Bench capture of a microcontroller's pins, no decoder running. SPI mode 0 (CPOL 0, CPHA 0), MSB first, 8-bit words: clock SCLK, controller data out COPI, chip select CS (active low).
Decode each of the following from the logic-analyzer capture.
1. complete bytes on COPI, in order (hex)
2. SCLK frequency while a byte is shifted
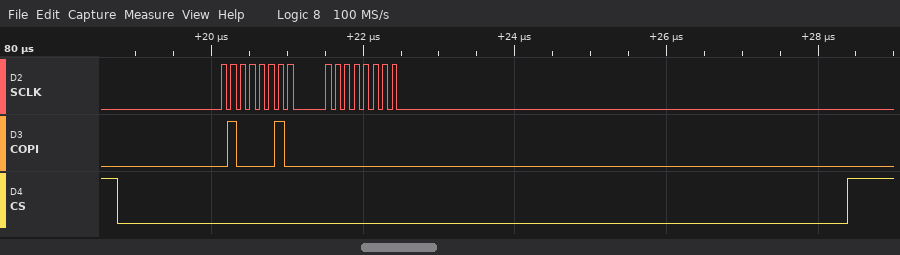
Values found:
42 00
8 MHz
